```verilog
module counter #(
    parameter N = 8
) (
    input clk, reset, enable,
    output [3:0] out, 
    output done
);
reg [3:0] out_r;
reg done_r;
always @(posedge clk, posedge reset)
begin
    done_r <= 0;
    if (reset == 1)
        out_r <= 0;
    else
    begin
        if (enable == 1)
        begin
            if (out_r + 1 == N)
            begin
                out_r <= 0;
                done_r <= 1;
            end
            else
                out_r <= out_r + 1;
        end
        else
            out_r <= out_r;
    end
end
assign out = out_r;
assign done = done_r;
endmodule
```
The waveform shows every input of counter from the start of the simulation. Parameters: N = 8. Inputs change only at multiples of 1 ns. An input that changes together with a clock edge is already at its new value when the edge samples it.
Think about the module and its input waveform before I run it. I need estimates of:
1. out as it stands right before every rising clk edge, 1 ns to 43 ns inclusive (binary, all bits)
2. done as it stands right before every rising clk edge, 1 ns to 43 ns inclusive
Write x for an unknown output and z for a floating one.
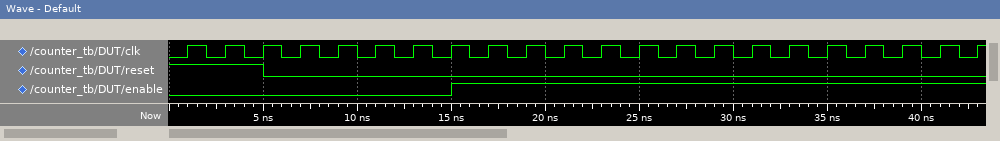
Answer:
0000, 0000, 0000, 0000, 0000, 0000, 0000, 0000, 0001, 0010, 0011, 0100, 0101, 0110, 0111, 0000, 0001, 0010, 0011, 0100, 0101, 0110
0 0 0 0 0 0 0 0 0 0 0 0 0 0 0 1 0 0 0 0 0 0
